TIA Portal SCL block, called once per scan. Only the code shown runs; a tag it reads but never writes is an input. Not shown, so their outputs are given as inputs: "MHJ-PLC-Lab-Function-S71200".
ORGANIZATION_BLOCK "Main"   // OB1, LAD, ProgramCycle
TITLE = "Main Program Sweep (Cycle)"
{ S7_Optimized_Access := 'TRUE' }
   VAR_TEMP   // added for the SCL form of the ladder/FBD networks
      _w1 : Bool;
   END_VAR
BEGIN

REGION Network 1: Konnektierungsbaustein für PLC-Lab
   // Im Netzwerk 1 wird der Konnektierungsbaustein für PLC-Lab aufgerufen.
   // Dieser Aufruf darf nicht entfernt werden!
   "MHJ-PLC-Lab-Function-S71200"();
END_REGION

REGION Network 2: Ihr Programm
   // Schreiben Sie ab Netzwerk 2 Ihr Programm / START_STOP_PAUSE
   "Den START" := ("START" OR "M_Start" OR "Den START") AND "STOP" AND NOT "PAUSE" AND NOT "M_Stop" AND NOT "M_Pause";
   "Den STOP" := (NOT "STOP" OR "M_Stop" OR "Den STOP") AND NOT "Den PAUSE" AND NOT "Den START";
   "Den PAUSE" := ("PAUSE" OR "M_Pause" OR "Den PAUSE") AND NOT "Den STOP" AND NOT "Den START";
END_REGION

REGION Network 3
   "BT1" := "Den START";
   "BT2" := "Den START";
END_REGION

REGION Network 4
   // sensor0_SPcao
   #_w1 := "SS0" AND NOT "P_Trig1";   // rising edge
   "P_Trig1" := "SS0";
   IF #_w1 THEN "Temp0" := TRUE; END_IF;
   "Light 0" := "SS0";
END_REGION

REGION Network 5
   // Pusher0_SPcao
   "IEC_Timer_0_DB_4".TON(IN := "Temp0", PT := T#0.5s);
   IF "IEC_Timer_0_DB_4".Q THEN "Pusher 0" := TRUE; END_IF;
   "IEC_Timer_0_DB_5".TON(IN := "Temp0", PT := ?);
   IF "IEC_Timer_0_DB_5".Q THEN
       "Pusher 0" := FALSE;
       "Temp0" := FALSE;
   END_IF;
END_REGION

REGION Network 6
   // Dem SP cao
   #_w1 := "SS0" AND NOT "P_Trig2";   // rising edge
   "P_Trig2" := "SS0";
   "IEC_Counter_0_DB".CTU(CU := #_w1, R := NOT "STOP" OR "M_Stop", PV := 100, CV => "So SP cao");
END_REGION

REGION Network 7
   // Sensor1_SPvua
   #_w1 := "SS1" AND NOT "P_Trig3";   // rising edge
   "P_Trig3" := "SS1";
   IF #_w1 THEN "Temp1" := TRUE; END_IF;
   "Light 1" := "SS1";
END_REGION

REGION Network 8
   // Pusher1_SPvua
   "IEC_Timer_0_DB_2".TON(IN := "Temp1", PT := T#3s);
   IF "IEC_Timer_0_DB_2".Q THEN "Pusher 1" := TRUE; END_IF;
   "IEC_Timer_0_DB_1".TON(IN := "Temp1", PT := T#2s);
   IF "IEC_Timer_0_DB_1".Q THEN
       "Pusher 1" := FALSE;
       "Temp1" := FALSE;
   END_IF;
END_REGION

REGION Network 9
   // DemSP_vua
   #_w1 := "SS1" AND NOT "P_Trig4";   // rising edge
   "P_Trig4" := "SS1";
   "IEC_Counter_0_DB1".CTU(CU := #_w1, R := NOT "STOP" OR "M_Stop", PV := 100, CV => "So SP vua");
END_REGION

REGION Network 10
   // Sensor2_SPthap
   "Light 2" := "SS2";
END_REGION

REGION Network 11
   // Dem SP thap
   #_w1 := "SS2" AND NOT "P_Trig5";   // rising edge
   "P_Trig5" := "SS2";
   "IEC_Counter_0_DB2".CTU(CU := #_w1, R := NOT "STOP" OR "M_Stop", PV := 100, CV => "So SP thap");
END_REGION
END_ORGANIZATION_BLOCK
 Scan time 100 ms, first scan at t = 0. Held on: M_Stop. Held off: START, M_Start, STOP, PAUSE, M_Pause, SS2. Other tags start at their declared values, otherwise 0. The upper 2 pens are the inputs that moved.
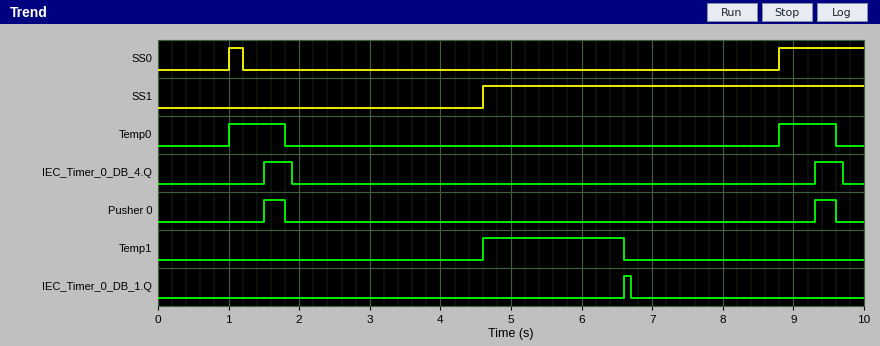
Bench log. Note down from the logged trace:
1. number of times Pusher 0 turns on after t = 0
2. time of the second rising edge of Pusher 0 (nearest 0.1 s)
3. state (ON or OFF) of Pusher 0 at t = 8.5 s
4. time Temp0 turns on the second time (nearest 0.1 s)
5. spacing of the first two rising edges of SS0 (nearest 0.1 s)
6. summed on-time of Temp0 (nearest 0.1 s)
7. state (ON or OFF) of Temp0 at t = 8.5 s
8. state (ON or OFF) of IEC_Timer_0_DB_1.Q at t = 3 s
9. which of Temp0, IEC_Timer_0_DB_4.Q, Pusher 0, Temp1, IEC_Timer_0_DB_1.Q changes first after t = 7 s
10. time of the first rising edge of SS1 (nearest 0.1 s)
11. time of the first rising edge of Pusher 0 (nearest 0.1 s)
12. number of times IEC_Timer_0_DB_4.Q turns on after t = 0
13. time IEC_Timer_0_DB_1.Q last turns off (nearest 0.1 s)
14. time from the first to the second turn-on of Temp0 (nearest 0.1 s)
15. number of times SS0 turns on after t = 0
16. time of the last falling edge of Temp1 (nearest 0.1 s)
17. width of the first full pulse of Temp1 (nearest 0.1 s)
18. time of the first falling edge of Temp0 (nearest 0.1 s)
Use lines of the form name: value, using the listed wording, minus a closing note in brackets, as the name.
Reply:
number of times Pusher 0 turns on after t = 0: 2
time of the second rising edge of Pusher 0: 9.3 s
state (ON or OFF) of Pusher 0 at t = 8.5 s: OFF
time Temp0 turns on the second time: 8.8 s
spacing of the first two rising edges of SS0: 7.8 s
summed on-time of Temp0: 1.6 s
state (ON or OFF) of Temp0 at t = 8.5 s: OFF
state (ON or OFF) of IEC_Timer_0_DB_1.Q at t = 3 s: OFF
which of Temp0, IEC_Timer_0_DB_4.Q, Pusher 0, Temp1, IEC_Timer_0_DB_1.Q changes first after t = 7 s: Temp0
time of the first rising edge of SS1: 4.6 s
time of the first rising edge of Pusher 0: 1.5 s
number of times IEC_Timer_0_DB_4.Q turns on after t = 0: 2
time IEC_Timer_0_DB_1.Q last turns off: 6.7 s
time from the first to the second turn-on of Temp0: 7.8 s
number of times SS0 turns on after t = 0: 2
time of the last falling edge of Temp1: 6.6 s
width of the first full pulse of Temp1: 2.0 s
time of the first falling edge of Temp0: 1.8 s
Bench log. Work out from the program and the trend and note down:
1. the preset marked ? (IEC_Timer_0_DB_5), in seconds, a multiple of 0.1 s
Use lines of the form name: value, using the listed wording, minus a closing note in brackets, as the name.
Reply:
the preset marked ? (IEC_Timer_0_DB_5), in seconds, a multiple of 0.1 s: 0.8 s
